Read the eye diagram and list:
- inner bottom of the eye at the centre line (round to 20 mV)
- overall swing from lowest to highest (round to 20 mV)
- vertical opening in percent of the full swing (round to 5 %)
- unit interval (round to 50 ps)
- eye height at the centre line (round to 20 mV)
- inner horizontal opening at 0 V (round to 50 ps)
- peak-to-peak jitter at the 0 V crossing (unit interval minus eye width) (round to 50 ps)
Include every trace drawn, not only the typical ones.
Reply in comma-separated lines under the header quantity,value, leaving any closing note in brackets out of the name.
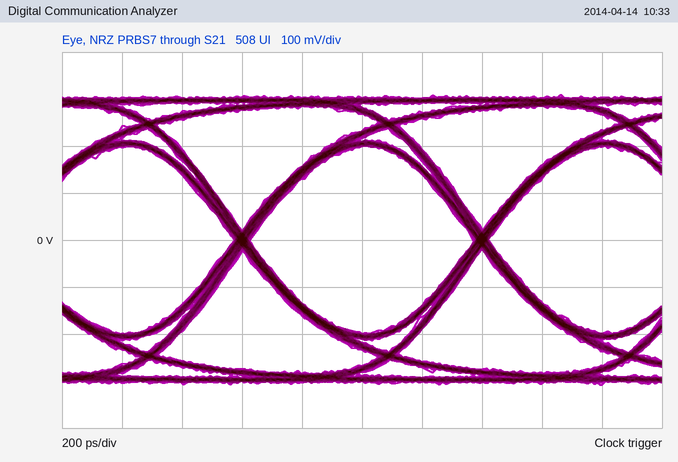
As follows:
quantity,value
inner bottom of the eye at the centre line,-200 mV
overall swing from lowest to highest,620 mV
vertical opening in percent of the full swing,65 %
unit interval,800 ps
eye height at the centre line,400 mV
inner horizontal opening at 0 V,750 ps
peak-to-peak jitter at the 0 V crossing (unit interval minus eye width),50 ps
